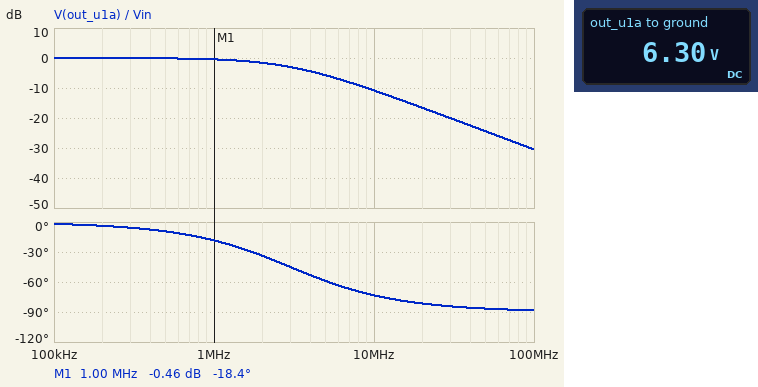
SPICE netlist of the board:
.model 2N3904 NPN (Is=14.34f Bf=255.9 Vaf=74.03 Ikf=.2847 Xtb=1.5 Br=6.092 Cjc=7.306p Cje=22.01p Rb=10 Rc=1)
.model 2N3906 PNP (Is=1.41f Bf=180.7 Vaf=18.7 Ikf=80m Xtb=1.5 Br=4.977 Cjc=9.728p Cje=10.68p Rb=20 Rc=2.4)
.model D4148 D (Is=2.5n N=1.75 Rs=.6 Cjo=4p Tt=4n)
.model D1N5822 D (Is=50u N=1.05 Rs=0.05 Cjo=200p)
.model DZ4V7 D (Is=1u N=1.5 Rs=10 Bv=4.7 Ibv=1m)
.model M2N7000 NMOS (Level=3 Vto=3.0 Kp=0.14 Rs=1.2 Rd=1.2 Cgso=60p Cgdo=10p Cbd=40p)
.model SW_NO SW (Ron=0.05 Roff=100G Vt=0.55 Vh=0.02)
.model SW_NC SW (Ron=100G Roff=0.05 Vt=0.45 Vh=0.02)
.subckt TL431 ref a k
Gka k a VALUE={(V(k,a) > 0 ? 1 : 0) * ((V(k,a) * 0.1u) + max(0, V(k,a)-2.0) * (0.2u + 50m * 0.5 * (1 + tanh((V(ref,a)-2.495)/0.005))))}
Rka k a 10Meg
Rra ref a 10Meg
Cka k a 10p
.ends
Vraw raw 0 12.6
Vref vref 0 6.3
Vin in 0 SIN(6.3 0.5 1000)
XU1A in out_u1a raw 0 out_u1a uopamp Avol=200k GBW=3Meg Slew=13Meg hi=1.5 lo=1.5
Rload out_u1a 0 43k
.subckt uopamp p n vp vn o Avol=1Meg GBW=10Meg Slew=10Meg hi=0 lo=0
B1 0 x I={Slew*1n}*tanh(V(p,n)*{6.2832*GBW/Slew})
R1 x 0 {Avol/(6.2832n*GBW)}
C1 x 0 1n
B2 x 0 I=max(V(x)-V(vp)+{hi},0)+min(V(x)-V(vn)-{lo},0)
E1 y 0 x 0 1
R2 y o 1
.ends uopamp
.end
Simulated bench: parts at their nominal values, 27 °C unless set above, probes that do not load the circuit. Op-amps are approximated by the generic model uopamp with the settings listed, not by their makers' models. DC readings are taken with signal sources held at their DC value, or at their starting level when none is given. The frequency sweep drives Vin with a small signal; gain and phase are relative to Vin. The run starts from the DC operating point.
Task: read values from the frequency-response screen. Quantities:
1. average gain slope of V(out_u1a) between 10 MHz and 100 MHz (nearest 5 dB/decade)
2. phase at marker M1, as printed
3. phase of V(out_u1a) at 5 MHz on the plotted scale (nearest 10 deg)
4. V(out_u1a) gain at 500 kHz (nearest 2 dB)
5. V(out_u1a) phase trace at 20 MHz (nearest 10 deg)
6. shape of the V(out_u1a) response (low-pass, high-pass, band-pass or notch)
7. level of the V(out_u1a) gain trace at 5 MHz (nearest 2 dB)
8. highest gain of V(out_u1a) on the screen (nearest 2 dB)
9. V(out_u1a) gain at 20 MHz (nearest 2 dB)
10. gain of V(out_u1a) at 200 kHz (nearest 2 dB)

-20 dB/decade
-18.4 deg
-60 deg
0 dB
-80 deg
low-pass
-6 dB
0 dB
-16 dB
0 dB
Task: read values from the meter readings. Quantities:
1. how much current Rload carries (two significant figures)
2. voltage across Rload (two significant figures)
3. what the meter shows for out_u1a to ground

150 µA
6.3 V
6.30 V
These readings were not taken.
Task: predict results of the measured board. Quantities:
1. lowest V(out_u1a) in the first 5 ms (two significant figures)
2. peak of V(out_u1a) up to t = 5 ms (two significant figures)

5.8 V
6.8 V
